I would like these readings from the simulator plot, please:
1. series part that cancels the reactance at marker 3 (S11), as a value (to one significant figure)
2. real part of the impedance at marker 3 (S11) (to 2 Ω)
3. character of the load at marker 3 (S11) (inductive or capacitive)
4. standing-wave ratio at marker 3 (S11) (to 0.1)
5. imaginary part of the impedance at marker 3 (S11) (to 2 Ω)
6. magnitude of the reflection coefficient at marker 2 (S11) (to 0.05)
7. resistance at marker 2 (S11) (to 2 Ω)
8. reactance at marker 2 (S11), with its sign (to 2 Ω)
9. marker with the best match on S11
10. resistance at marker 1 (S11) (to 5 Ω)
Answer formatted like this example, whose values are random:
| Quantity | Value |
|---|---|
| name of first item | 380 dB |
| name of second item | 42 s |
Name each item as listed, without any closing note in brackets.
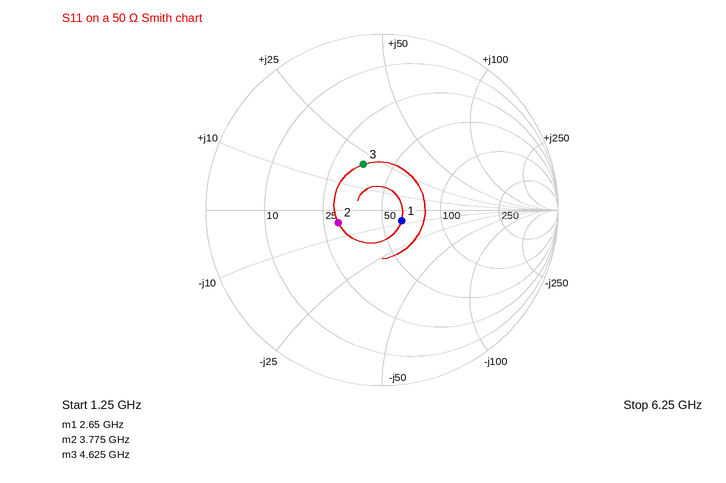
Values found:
| Quantity | Value |
|---|---|
| series part that cancels the reactance at marker 3 (S11), as a value | 2 pF |
| real part of the impedance at marker 3 (S11) | 36 Ω |
| character of the load at marker 3 (S11) | inductive |
| standing-wave ratio at marker 3 (S11) | 1.8 |
| imaginary part of the impedance at marker 3 (S11) | +20 Ω |
| magnitude of the reflection coefficient at marker 2 (S11) | 0.25 |
| resistance at marker 2 (S11) | 30 Ω |
| reactance at marker 2 (S11), with its sign | -4 Ω |
| marker with the best match on S11 | marker 1 |
| resistance at marker 1 (S11) | 60 Ω |
